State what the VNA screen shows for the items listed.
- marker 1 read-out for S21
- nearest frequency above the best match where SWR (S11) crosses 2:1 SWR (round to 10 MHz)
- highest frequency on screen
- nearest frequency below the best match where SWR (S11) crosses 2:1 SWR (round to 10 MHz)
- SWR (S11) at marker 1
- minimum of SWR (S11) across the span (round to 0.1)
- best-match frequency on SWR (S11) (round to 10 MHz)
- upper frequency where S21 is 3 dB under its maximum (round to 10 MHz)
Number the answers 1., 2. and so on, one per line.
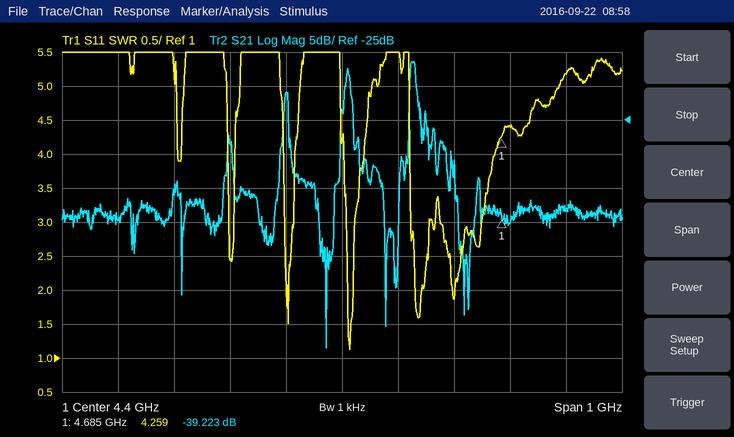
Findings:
1. -39.223 dB
2. 4.42 GHz
3. 4.9 GHz
4. 4.41 GHz
5. 4.259
6. 1.1
7. 4.41 GHz
8. 4.53 GHz
